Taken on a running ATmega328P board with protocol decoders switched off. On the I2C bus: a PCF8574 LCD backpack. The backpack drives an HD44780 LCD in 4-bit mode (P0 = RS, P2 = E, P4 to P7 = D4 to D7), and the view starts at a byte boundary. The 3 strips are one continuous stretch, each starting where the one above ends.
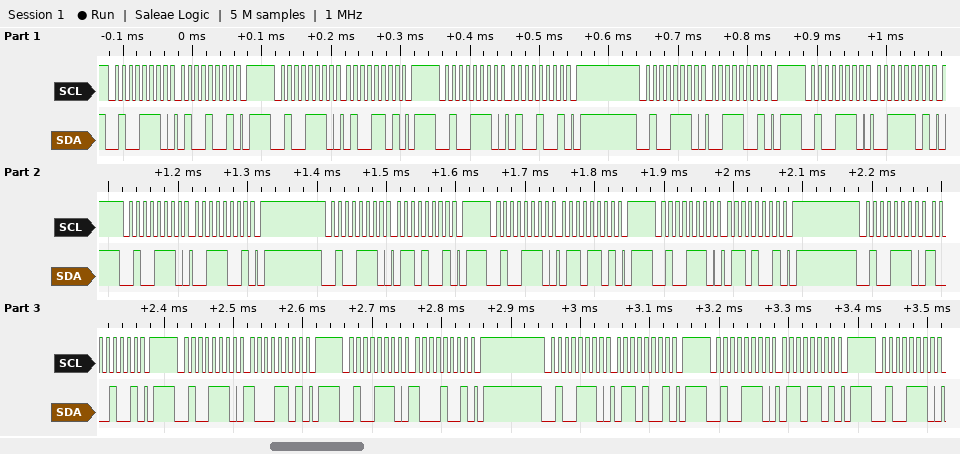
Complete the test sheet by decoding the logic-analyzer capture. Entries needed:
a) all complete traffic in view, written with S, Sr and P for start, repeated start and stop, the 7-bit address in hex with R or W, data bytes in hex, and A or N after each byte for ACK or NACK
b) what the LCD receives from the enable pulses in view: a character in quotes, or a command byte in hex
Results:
S 27W A 49 A P S 27W A 4D A P S 27W A 49 A P S 27W A 39 A P S 27W A 3D A P S 27W A 39 A P S 27W A 69 A P S 27W A 6D A P S 27W A 69 A P S 27W A 89 A P S 27W A 8D A P S 27W A 89 A P S 27W A 69 A P S 27W A 6D A P S 27W A
'C' 'h'
